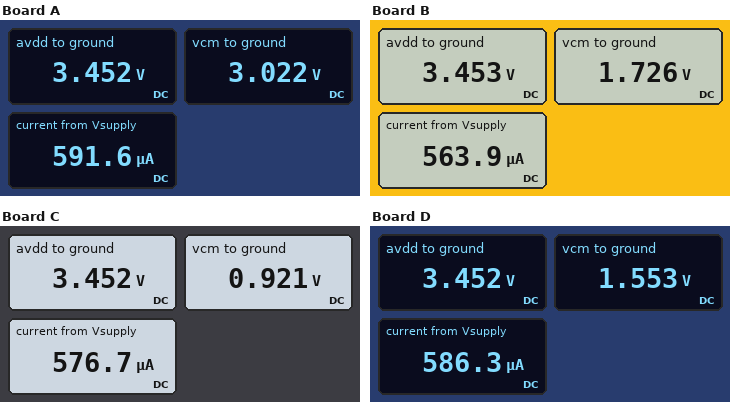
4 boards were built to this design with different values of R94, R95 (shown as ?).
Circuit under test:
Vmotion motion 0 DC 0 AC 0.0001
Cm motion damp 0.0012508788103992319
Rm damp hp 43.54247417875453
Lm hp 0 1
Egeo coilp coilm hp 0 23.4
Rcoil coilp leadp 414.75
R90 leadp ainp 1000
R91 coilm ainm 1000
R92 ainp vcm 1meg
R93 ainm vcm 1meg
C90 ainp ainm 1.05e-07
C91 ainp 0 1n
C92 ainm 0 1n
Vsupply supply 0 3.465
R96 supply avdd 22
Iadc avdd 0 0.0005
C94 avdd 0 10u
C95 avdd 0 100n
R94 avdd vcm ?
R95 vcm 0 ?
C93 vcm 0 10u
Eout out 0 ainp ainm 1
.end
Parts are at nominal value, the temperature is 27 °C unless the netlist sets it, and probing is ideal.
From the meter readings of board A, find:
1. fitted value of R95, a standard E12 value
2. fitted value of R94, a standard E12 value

33 kΩ
4.7 kΩ
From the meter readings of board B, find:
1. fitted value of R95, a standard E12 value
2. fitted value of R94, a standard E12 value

27 kΩ
27 kΩ
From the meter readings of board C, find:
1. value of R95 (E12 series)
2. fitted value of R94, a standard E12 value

12 kΩ
33 kΩ
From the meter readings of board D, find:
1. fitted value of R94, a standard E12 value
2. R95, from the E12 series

22 kΩ
18 kΩ
